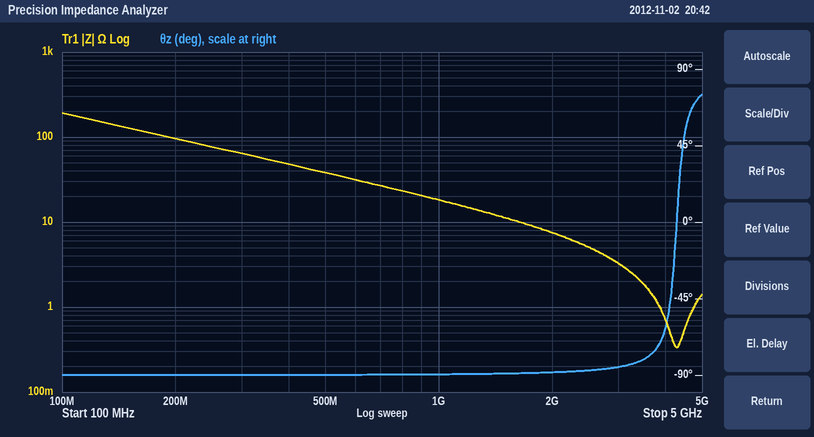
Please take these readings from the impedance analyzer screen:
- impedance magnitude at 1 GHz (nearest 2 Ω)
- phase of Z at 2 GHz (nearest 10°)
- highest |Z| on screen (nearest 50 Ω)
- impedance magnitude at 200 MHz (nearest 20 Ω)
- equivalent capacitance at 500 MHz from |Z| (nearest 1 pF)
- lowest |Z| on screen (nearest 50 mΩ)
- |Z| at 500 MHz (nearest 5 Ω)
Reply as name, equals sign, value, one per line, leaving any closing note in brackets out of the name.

impedance magnitude at 1 GHz = 18 Ω
phase of Z at 2 GHz = -90°
highest |Z| on screen = 200 Ω
impedance magnitude at 200 MHz = 100 Ω
equivalent capacitance at 500 MHz from |Z| = 8 pF
lowest |Z| on screen = 350 mΩ
|Z| at 500 MHz = 40 Ω
